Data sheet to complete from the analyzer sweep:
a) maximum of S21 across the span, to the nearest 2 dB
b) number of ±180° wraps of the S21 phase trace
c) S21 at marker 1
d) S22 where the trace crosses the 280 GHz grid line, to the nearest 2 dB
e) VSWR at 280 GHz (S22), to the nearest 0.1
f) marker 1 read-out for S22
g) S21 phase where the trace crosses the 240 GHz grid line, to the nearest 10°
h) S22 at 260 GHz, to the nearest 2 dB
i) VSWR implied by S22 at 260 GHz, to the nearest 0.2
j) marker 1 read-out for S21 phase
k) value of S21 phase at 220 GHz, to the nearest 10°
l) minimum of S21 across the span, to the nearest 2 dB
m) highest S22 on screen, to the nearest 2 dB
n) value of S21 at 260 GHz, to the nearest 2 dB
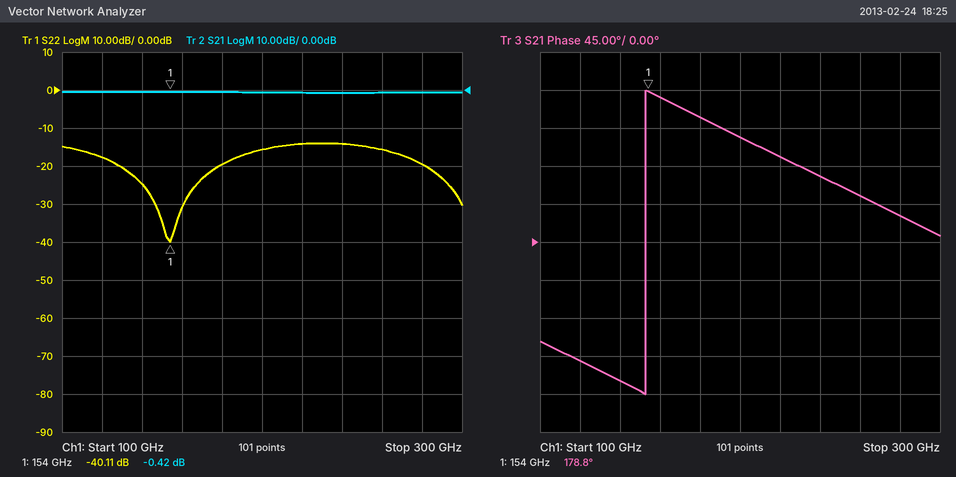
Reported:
0 dB
1
-0.42 dB
-20 dB
1.2
-40.11 dB
80°
-16 dB
1.4
178.8°
100°
0 dB
-14 dB
0 dB
